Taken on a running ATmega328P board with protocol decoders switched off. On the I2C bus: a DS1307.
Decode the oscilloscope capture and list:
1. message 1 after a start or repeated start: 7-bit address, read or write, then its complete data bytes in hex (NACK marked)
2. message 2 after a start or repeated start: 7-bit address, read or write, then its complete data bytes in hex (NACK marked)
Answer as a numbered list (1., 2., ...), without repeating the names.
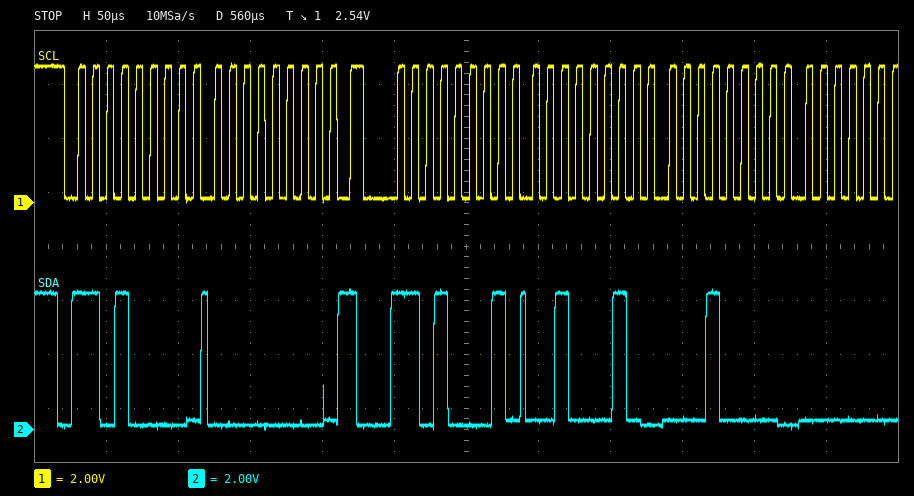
1. 0x68 write: 00
2. 0x68 read: 22 10
